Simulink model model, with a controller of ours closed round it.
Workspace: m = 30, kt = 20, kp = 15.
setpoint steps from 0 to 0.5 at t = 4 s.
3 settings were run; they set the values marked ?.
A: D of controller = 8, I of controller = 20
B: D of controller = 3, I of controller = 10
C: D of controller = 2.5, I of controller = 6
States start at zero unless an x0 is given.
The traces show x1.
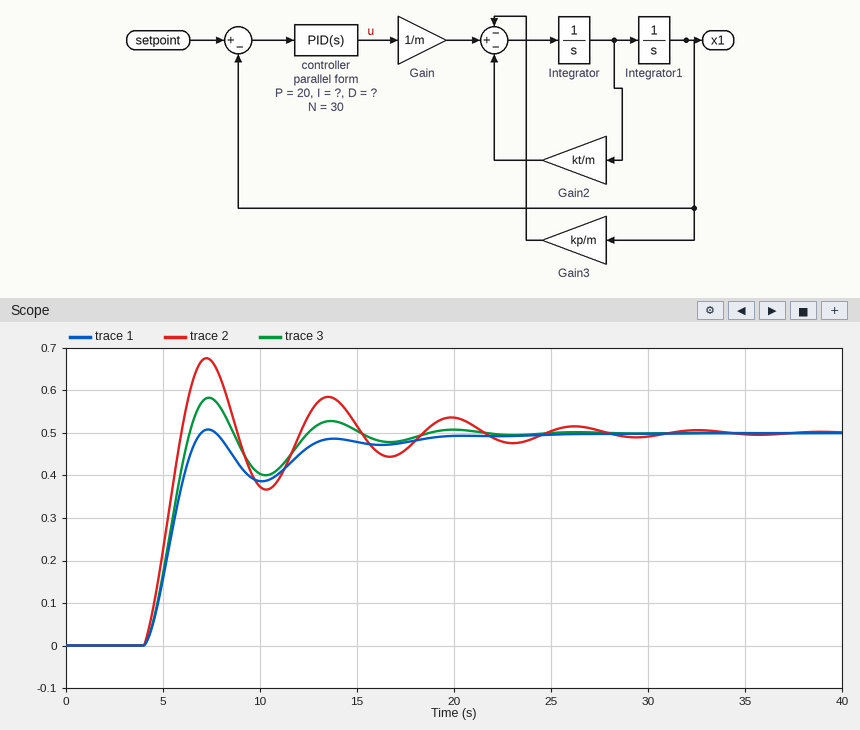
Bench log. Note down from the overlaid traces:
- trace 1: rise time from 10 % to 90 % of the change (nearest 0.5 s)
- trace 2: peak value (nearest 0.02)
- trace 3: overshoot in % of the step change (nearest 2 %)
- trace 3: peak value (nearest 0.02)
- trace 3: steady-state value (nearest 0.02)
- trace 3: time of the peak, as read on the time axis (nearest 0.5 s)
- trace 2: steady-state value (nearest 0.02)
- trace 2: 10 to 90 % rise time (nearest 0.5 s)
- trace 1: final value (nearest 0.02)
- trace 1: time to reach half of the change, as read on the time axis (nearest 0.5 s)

2.0 s
0.68
16 %
0.58
0.50
7.5 s
0.50
1.5 s
0.50
5.5 s
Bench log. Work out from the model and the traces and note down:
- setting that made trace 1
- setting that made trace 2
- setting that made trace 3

C
A
B
